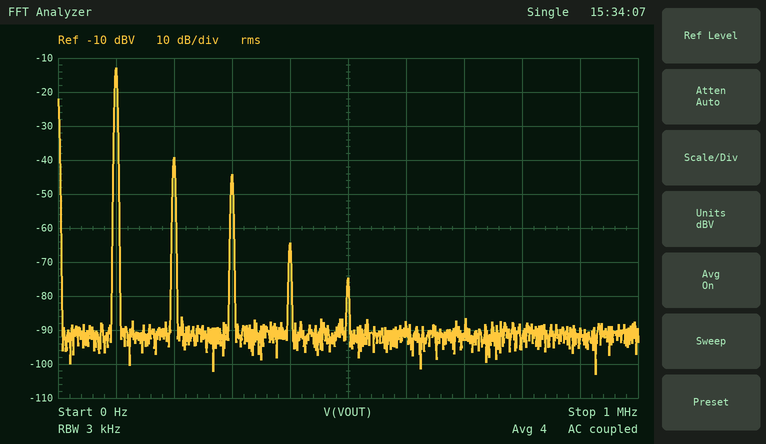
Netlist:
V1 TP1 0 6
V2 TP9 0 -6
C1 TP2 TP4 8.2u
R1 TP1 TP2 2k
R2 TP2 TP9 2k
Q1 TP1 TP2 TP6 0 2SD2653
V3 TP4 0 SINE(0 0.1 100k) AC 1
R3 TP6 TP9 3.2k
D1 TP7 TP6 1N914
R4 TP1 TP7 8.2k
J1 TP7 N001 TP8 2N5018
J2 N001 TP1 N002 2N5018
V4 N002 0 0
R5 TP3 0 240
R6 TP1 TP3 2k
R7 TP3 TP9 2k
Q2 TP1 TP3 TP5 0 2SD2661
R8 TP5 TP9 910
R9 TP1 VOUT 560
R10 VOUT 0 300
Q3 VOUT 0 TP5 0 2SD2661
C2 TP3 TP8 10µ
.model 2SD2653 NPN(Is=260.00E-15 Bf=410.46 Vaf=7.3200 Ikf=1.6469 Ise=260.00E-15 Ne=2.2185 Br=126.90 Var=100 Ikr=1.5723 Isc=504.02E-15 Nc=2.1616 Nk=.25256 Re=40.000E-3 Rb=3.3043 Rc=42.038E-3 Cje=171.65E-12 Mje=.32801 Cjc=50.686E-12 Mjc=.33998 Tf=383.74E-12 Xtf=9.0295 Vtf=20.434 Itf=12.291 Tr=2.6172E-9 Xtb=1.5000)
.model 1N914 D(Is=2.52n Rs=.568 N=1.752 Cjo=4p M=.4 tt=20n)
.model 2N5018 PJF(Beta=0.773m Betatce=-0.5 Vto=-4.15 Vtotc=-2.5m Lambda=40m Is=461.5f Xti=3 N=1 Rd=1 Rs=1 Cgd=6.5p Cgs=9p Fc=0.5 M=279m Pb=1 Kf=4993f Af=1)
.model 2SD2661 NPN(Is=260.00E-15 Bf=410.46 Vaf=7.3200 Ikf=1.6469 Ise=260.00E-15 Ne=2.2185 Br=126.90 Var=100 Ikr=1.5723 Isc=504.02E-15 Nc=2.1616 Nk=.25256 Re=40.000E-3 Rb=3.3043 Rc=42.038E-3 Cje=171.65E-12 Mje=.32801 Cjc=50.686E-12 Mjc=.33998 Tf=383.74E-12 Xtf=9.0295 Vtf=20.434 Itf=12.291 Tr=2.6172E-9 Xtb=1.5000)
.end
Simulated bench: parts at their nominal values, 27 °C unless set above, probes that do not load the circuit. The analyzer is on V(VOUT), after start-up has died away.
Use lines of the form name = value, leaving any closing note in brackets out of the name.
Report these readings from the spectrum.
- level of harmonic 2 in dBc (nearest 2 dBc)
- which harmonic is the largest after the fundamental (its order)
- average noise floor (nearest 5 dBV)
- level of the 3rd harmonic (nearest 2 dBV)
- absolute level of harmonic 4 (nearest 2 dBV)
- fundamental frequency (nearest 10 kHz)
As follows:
level of harmonic 2 in dBc = -26 dBc
which harmonic is the largest after the fundamental = 2
average noise floor = -90 dBV
level of the 3rd harmonic = -44 dBV
absolute level of harmonic 4 = -64 dBV
fundamental frequency = 100 kHz
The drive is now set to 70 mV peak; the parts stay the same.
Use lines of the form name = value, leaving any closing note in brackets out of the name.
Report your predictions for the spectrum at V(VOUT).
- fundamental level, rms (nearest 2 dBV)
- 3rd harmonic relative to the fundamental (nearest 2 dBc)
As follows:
fundamental level, rms = -16 dBV
3rd harmonic relative to the fundamental = -38 dBc
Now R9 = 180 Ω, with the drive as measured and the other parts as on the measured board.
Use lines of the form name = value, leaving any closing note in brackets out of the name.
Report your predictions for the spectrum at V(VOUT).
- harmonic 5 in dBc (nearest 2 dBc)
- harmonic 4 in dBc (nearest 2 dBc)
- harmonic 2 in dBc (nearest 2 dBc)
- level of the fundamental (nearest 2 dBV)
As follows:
harmonic 5 in dBc = -60 dBc
harmonic 4 in dBc = -56 dBc
harmonic 2 in dBc = -32 dBc
level of the fundamental = -18 dBV
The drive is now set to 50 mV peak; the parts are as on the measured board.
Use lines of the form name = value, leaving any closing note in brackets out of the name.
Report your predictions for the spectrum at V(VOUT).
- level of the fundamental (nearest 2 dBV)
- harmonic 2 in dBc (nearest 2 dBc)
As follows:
level of the fundamental = -18 dBV
harmonic 2 in dBc = -32 dBc
